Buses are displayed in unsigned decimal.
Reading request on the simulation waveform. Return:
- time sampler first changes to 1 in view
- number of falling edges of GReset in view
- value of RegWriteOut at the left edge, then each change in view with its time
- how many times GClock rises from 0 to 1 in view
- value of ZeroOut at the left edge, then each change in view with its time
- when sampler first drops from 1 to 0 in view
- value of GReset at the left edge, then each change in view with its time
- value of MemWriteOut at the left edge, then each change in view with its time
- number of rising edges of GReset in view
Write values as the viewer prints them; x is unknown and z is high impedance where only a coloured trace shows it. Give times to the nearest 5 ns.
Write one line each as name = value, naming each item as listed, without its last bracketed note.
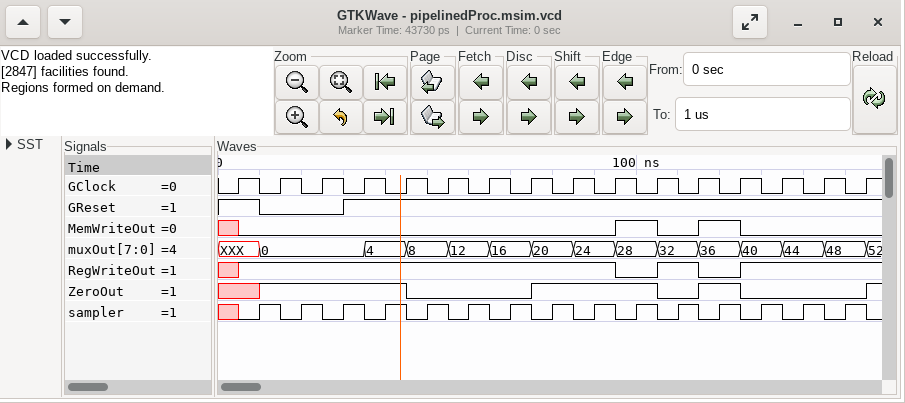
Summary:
time sampler first changes to 1 in view = 10 ns
number of falling edges of GReset in view = 1
value of RegWriteOut at the left edge, then each change in view with its time = x, 1 at 5 ns, 0 at 95 ns, 1 at 105 ns, 0 at 115 ns, 1 at 125 ns
how many times GClock rises from 0 to 1 in view = 16
value of ZeroOut at the left edge, then each change in view with its time = x, 1 at 10 ns, 0 at 45 ns, 1 at 75 ns, 0 at 105 ns, 1 at 115 ns, 0 at 125 ns, 1 at 155 ns
when sampler first drops from 1 to 0 in view = 15 ns
value of GReset at the left edge, then each change in view with its time = 1, 0 at 10 ns, 1 at 30 ns
value of MemWriteOut at the left edge, then each change in view with its time = x, 0 at 5 ns, 1 at 95 ns, 0 at 105 ns, 1 at 115 ns, 0 at 125 ns
number of rising edges of GReset in view = 1
